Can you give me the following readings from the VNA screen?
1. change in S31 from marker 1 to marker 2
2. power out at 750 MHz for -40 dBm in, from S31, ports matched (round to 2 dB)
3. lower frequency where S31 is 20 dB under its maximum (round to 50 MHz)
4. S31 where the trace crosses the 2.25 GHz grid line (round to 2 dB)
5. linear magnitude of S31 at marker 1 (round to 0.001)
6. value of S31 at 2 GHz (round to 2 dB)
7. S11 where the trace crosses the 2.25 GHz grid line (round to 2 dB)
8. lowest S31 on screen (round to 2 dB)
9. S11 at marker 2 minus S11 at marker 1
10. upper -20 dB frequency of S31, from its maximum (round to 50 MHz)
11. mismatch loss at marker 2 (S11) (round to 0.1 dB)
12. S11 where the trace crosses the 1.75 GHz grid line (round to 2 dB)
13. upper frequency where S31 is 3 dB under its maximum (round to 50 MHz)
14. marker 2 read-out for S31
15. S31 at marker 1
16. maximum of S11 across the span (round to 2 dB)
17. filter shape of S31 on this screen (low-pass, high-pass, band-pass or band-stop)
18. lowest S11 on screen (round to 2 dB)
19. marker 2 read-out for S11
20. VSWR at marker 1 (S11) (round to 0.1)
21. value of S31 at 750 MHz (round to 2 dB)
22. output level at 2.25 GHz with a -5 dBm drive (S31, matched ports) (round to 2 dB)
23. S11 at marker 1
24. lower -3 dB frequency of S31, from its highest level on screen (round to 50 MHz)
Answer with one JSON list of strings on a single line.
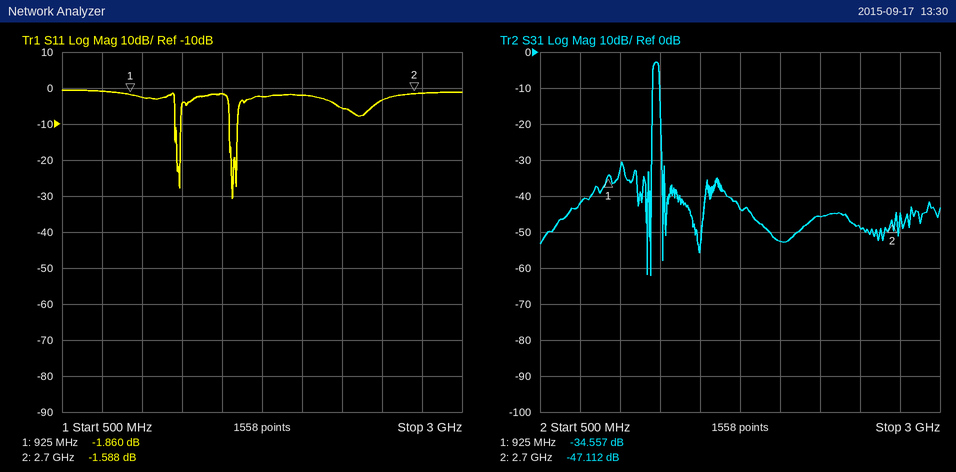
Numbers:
["-12.555 dB", "-82 dBm", "1.20 GHz", "-46 dB", "0.019", "-52 dB", "-6 dB", "-62 dB", "0.272 dB", "1.25 GHz", "5.1 dB", "-2 dB", "1.25 GHz", "-47.112 dB", "-34.557 dB", "0 dB", "band-pass", "-30 dB", "-1.588 dB", "9.4", "-42 dB", "-50 dBm", "-1.860 dB", "1.20 GHz"]
